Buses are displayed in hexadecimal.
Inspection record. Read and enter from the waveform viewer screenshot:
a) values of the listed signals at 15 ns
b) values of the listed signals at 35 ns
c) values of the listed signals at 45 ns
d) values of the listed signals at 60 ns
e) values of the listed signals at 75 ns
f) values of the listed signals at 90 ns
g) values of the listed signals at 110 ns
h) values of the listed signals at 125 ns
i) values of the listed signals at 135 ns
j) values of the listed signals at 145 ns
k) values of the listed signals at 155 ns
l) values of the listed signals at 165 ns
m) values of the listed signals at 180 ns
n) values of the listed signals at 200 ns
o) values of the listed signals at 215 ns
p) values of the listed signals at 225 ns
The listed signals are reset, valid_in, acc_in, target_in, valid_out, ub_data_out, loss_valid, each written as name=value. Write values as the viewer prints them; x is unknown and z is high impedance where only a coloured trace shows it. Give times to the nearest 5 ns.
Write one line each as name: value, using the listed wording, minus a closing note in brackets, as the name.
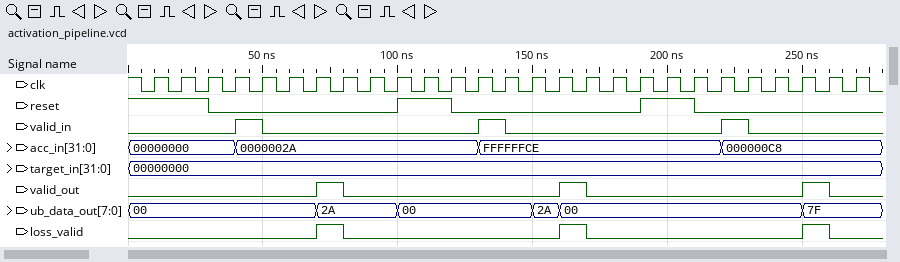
values of the listed signals at 15 ns: reset=1, valid_in=0, acc_in=00000000, target_in=00000000, valid_out=0, ub_data_out=00, loss_valid=0
values of the listed signals at 35 ns: reset=0, valid_in=0, acc_in=00000000, target_in=00000000, valid_out=0, ub_data_out=00, loss_valid=0
values of the listed signals at 45 ns: reset=0, valid_in=1, acc_in=0000002A, target_in=00000000, valid_out=0, ub_data_out=00, loss_valid=0
values of the listed signals at 60 ns: reset=0, valid_in=0, acc_in=0000002A, target_in=00000000, valid_out=0, ub_data_out=00, loss_valid=0
values of the listed signals at 75 ns: reset=0, valid_in=0, acc_in=0000002A, target_in=00000000, valid_out=1, ub_data_out=2A, loss_valid=1
values of the listed signals at 90 ns: reset=0, valid_in=0, acc_in=0000002A, target_in=00000000, valid_out=0, ub_data_out=2A, loss_valid=0
values of the listed signals at 110 ns: reset=1, valid_in=0, acc_in=0000002A, target_in=00000000, valid_out=0, ub_data_out=00, loss_valid=0
values of the listed signals at 125 ns: reset=0, valid_in=0, acc_in=0000002A, target_in=00000000, valid_out=0, ub_data_out=00, loss_valid=0
values of the listed signals at 135 ns: reset=0, valid_in=1, acc_in=FFFFFFCE, target_in=00000000, valid_out=0, ub_data_out=00, loss_valid=0
values of the listed signals at 145 ns: reset=0, valid_in=0, acc_in=FFFFFFCE, target_in=00000000, valid_out=0, ub_data_out=00, loss_valid=0
values of the listed signals at 155 ns: reset=0, valid_in=0, acc_in=FFFFFFCE, target_in=00000000, valid_out=0, ub_data_out=2A, loss_valid=0
values of the listed signals at 165 ns: reset=0, valid_in=0, acc_in=FFFFFFCE, target_in=00000000, valid_out=1, ub_data_out=00, loss_valid=1
values of the listed signals at 180 ns: reset=0, valid_in=0, acc_in=FFFFFFCE, target_in=00000000, valid_out=0, ub_data_out=00, loss_valid=0
values of the listed signals at 200 ns: reset=1, valid_in=0, acc_in=FFFFFFCE, target_in=00000000, valid_out=0, ub_data_out=00, loss_valid=0
values of the listed signals at 215 ns: reset=0, valid_in=0, acc_in=FFFFFFCE, target_in=00000000, valid_out=0, ub_data_out=00, loss_valid=0
values of the listed signals at 225 ns: reset=0, valid_in=1, acc_in=000000C8, target_in=00000000, valid_out=0, ub_data_out=00, loss_valid=0
